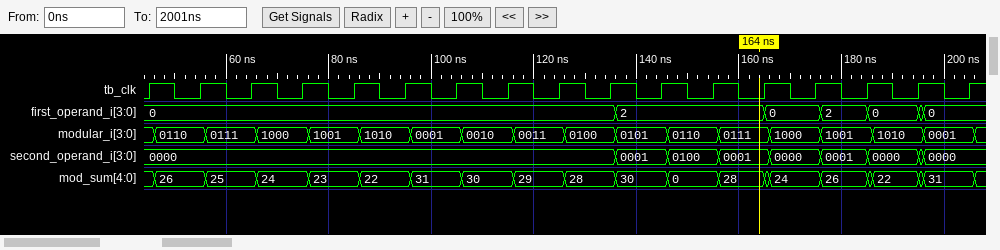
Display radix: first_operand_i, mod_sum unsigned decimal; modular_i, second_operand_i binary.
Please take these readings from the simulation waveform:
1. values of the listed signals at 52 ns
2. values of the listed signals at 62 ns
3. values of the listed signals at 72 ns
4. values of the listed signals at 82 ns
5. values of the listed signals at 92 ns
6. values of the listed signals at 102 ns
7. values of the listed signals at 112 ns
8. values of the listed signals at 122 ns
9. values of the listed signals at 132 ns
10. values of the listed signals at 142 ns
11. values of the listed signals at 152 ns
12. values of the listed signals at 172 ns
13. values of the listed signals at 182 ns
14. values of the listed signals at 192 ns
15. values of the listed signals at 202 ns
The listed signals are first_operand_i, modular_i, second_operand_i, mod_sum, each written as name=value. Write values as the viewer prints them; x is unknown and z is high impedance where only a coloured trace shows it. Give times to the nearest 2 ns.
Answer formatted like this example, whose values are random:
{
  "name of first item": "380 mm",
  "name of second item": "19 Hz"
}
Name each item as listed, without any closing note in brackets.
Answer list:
{
  "values of the listed signals at 52 ns": "first_operand_i=0, modular_i=0110, second_operand_i=0000, mod_sum=26",
  "values of the listed signals at 62 ns": "first_operand_i=0, modular_i=0111, second_operand_i=0000, mod_sum=25",
  "values of the listed signals at 72 ns": "first_operand_i=0, modular_i=1000, second_operand_i=0000, mod_sum=24",
  "values of the listed signals at 82 ns": "first_operand_i=0, modular_i=1001, second_operand_i=0000, mod_sum=23",
  "values of the listed signals at 92 ns": "first_operand_i=0, modular_i=1010, second_operand_i=0000, mod_sum=22",
  "values of the listed signals at 102 ns": "first_operand_i=0, modular_i=0001, second_operand_i=0000, mod_sum=31",
  "values of the listed signals at 112 ns": "first_operand_i=0, modular_i=0010, second_operand_i=0000, mod_sum=30",
  "values of the listed signals at 122 ns": "first_operand_i=0, modular_i=0011, second_operand_i=0000, mod_sum=29",
  "values of the listed signals at 132 ns": "first_operand_i=0, modular_i=0100, second_operand_i=0000, mod_sum=28",
  "values of the listed signals at 142 ns": "first_operand_i=2, modular_i=0101, second_operand_i=0001, mod_sum=30",
  "values of the listed signals at 152 ns": "first_operand_i=2, modular_i=0110, second_operand_i=0100, mod_sum=0",
  "values of the listed signals at 172 ns": "first_operand_i=0, modular_i=1000, second_operand_i=0000, mod_sum=24",
  "values of the listed signals at 182 ns": "first_operand_i=2, modular_i=1001, second_operand_i=0001, mod_sum=26",
  "values of the listed signals at 192 ns": "first_operand_i=0, modular_i=1010, second_operand_i=0000, mod_sum=22",
  "values of the listed signals at 202 ns": "first_operand_i=0, modular_i=0001, second_operand_i=0000, mod_sum=31"
}
